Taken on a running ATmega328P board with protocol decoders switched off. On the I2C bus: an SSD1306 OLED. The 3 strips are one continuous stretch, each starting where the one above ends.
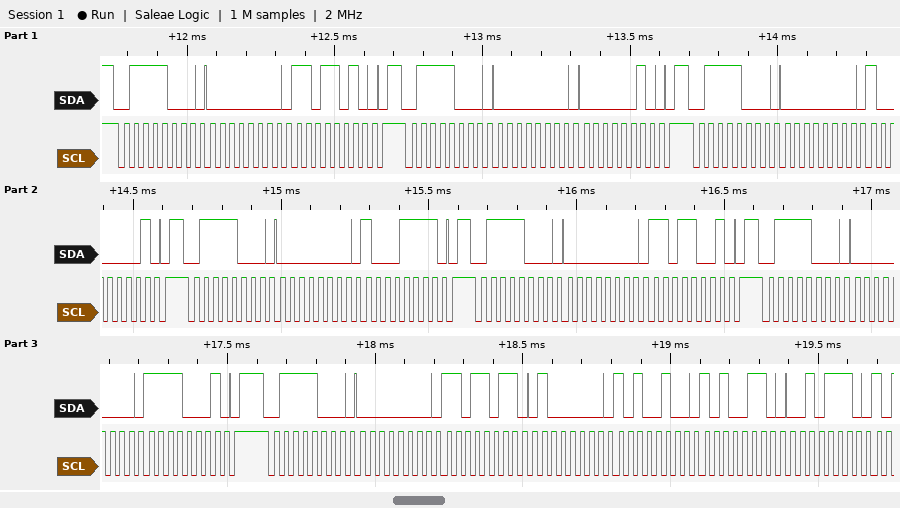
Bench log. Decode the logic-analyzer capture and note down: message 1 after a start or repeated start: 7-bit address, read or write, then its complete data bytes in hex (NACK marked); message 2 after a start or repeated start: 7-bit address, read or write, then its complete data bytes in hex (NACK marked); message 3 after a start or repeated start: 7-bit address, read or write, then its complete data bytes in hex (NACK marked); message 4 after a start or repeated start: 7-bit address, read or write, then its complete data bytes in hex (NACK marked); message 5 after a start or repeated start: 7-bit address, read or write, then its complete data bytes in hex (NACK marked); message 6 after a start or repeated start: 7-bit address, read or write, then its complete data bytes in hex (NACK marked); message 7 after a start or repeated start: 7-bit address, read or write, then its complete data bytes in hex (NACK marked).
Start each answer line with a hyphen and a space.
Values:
- 0x3C write: 00 DA
- 0x3C write: 00 02
- 0x3C write: 00 81
- 0x3C write: 00 8F
- 0x3C write: 00 D9
- 0x3C write: 00 F1
- 0x3C write: 00 DB 40 A4 A6 2E
